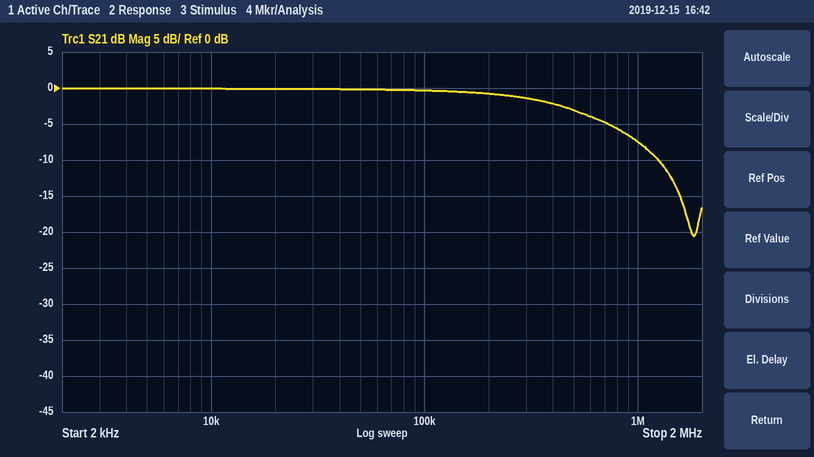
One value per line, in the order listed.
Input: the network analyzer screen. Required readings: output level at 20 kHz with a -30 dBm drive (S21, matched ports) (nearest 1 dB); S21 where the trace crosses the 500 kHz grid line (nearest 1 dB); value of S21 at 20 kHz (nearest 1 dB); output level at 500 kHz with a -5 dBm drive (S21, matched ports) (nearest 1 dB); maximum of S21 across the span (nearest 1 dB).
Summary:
-30 dBm
-3 dB
0 dB
-8 dBm
0 dB
